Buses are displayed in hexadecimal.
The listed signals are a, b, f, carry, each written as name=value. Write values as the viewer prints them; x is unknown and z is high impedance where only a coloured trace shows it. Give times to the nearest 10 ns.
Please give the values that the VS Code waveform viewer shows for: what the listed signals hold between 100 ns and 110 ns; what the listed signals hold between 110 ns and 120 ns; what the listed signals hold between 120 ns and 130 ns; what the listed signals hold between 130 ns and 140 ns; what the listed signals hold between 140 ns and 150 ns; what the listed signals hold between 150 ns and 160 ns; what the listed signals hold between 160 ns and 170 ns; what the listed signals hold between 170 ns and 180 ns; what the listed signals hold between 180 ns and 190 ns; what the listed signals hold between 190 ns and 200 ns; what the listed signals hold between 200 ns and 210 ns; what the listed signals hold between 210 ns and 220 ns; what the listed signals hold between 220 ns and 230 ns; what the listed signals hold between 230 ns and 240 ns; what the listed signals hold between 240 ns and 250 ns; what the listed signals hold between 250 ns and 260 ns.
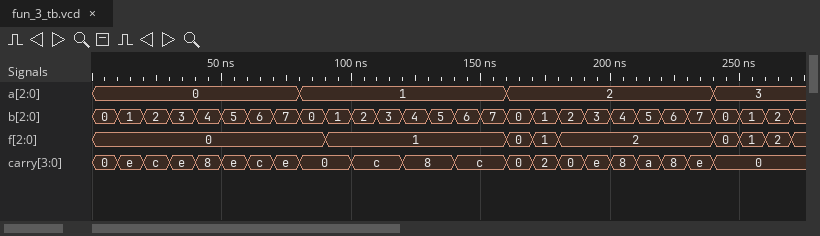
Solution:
a=1, b=2, f=1, carry=c
a=1, b=3, f=1, carry=c
a=1, b=4, f=1, carry=8
a=1, b=5, f=1, carry=8
a=1, b=6, f=1, carry=c
a=1, b=7, f=1, carry=c
a=2, b=0, f=0, carry=0
a=2, b=1, f=1, carry=2
a=2, b=2, f=2, carry=0
a=2, b=3, f=2, carry=e
a=2, b=4, f=2, carry=8
a=2, b=5, f=2, carry=a
a=2, b=6, f=2, carry=8
a=2, b=7, f=2, carry=e
a=3, b=0, f=0, carry=0
a=3, b=1, f=1, carry=0
